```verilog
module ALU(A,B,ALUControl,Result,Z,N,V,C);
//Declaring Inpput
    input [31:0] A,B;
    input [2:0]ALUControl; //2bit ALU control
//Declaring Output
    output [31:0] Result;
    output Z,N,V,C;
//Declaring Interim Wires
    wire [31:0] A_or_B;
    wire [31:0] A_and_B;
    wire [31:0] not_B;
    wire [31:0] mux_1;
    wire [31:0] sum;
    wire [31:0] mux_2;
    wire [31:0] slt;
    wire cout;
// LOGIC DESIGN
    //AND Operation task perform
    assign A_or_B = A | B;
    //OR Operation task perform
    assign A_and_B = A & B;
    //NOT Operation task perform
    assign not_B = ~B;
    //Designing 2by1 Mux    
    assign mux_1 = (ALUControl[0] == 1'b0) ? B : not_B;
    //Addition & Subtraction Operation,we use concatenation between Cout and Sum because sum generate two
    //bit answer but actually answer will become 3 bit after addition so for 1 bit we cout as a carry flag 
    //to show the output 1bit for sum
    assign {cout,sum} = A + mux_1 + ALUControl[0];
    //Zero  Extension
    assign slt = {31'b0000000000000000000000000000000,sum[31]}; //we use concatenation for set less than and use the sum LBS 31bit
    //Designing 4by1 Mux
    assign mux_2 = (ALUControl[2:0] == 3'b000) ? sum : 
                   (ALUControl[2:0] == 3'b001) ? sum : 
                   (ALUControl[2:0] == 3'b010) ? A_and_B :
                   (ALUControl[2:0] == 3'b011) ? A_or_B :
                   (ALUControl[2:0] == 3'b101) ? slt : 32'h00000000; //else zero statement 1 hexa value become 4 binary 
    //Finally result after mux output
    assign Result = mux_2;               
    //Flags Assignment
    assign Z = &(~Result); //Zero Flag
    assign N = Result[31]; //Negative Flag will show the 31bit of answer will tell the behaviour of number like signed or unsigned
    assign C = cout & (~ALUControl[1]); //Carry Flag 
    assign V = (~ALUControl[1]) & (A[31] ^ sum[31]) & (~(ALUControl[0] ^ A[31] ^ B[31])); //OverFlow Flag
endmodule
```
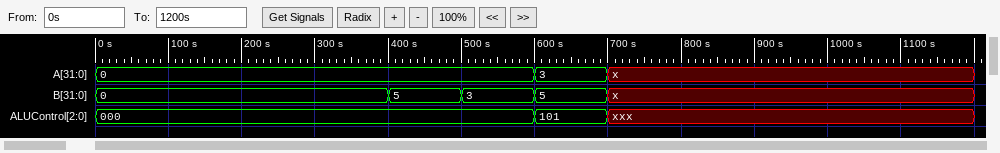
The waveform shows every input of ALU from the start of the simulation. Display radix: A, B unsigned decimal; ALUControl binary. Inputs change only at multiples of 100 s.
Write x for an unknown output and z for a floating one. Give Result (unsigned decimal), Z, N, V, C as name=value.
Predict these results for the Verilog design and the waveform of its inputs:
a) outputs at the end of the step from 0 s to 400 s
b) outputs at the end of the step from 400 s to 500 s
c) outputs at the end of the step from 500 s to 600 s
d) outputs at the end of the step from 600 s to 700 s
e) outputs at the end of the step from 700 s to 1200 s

Result=0, Z=1, N=0, V=0, C=0
Result=5, Z=0, N=0, V=0, C=0
Result=3, Z=0, N=0, V=0, C=0
Result=1, Z=0, N=0, V=0, C=0
Result=x, Z=x, N=x, V=x, C=x
